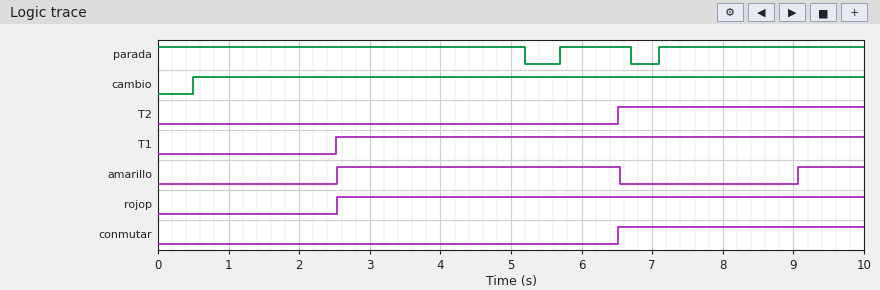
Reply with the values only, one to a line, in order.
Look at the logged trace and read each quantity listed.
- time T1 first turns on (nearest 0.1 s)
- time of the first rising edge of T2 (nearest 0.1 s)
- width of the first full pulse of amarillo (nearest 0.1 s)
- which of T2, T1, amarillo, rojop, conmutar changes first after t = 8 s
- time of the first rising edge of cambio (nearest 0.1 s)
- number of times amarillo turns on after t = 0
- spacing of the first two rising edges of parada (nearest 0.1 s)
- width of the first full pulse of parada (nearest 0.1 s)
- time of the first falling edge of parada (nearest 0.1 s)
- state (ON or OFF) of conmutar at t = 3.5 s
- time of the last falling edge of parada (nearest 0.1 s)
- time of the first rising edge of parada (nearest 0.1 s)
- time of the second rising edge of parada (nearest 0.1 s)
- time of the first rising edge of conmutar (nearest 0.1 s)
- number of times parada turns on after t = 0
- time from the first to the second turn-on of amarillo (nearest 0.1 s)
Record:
2.5 s
6.5 s
4.0 s
amarillo
0.5 s
2
1.4 s
1.0 s
5.2 s
OFF
6.7 s
5.7 s
7.1 s
6.5 s
2
6.5 s
